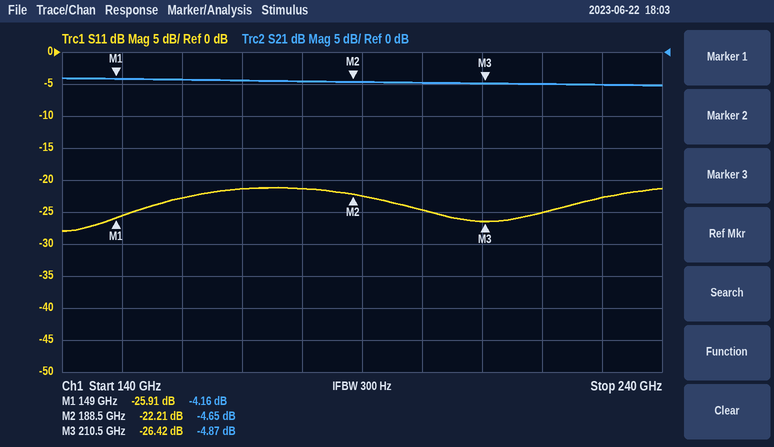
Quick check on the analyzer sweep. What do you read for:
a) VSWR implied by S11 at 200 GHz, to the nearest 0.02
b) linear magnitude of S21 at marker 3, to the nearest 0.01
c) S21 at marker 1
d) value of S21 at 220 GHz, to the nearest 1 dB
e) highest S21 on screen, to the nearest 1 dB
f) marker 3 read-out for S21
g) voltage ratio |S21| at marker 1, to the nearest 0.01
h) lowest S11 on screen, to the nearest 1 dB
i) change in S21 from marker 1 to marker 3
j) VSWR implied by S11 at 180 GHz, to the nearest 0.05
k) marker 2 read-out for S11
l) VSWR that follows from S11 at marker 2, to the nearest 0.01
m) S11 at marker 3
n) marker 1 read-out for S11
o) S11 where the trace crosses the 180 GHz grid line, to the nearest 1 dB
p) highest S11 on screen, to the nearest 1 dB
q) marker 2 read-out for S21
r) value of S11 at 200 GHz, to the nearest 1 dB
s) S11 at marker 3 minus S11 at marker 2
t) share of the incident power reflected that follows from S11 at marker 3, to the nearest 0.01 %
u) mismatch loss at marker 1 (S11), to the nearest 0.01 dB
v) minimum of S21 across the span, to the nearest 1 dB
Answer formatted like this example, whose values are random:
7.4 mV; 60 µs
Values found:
1.12; 0.57; -4.16 dB; -5 dB; -4 dB; -4.87 dB; 0.62; -28 dB; -0.71 dB; 1.20; -22.21 dB; 1.17; -26.42 dB; -25.91 dB; -21 dB; -21 dB; -4.65 dB; -25 dB; -4.21 dB; 0.23 %; 0.01 dB; -5 dB
